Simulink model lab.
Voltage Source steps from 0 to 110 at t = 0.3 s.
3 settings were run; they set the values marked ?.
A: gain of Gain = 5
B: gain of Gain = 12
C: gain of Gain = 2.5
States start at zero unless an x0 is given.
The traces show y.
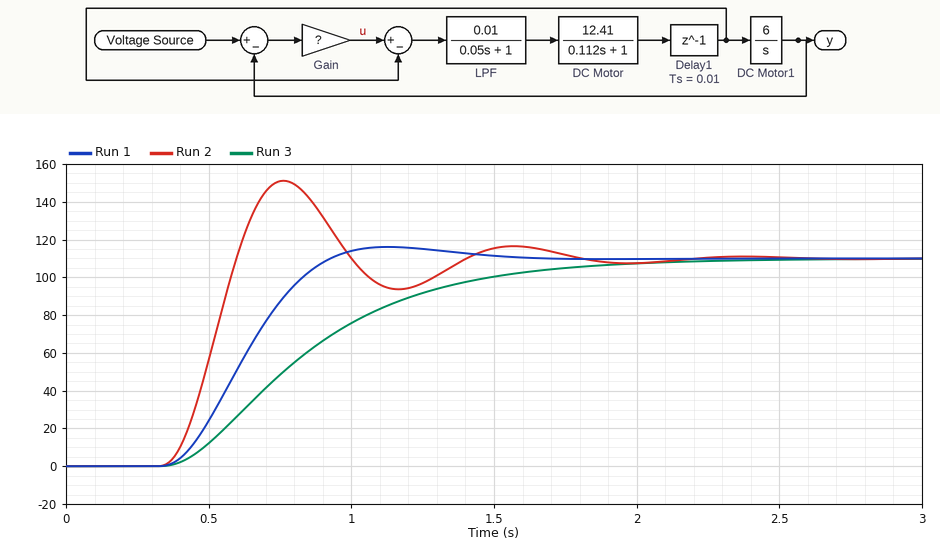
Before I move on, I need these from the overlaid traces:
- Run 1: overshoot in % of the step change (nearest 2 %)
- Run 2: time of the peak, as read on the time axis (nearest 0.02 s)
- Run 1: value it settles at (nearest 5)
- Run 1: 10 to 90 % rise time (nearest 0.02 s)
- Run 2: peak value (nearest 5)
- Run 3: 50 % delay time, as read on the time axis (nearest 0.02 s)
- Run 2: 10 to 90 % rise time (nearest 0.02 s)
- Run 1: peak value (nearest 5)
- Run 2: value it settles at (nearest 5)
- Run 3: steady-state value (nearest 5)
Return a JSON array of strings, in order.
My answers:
["6 %", "0.76 s", "110", "0.38 s", "150", "0.80 s", "0.18 s", "115", "110", "110"]
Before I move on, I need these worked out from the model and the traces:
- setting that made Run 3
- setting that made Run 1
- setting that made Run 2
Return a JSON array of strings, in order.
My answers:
["C", "A", "B"]
